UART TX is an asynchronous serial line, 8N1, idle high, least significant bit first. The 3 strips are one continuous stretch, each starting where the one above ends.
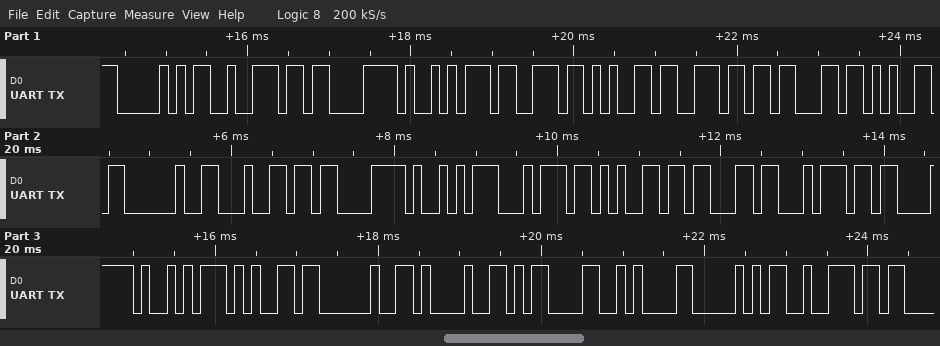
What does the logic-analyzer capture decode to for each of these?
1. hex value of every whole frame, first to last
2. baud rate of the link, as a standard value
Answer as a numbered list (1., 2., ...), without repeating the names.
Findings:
1. 50 72 C3 A9 73 65 6E 63 65 20 64 C3 A9 74 65 63 74 C3 A9 65 20 21 0D 0A 50 72
2. 9600 baud
